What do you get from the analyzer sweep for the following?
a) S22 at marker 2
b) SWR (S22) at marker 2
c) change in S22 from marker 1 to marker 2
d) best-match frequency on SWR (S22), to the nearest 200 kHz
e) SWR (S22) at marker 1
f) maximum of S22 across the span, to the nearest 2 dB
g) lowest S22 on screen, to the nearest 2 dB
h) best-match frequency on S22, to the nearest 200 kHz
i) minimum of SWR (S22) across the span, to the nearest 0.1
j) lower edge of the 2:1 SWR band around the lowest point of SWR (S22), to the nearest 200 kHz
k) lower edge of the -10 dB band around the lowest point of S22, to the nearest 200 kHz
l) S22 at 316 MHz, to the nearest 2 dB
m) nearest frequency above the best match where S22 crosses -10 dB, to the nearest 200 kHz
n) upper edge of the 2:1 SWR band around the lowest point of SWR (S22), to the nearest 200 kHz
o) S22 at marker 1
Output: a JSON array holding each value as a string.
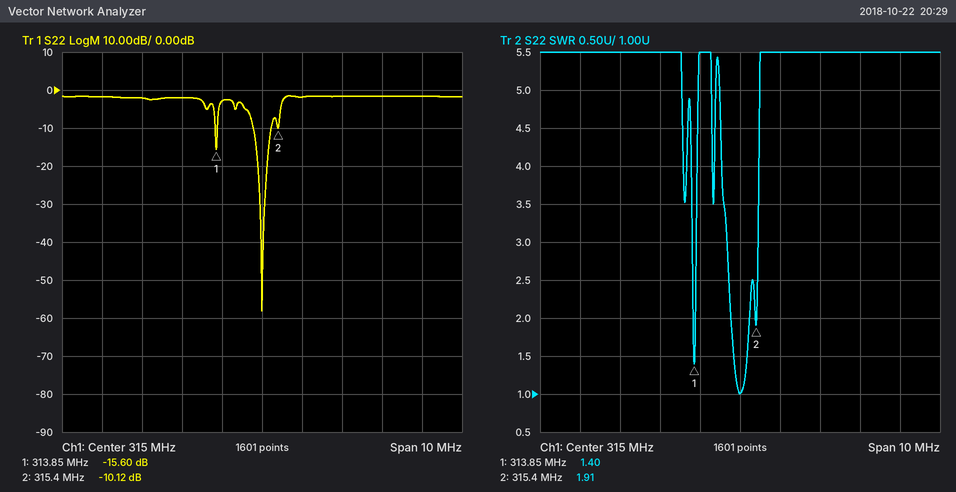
["-10.12 dB", "1.91", "5.48 dB", "315.0 MHz", "1.40", "-2 dB", "-58 dB", "315.0 MHz", "1.0", "314.8 MHz", "314.8 MHz", "-2 dB", "315.2 MHz", "315.2 MHz", "-15.60 dB"]
